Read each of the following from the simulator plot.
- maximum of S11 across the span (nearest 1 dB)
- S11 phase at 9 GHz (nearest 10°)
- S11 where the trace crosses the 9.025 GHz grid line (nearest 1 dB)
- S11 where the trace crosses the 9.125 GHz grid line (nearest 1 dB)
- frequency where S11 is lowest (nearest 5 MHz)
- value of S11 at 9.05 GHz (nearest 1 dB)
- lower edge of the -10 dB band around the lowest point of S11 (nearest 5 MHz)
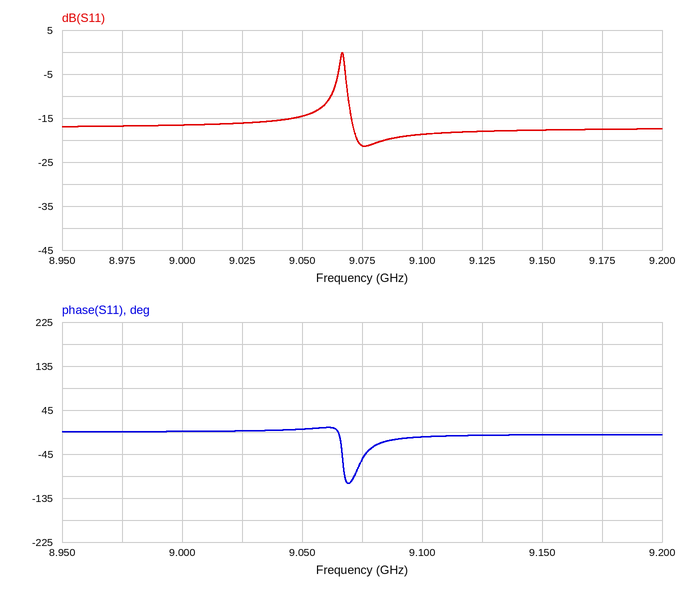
0 dB
0°
-16 dB
-18 dB
9.075 GHz
-15 dB
9.070 GHz
